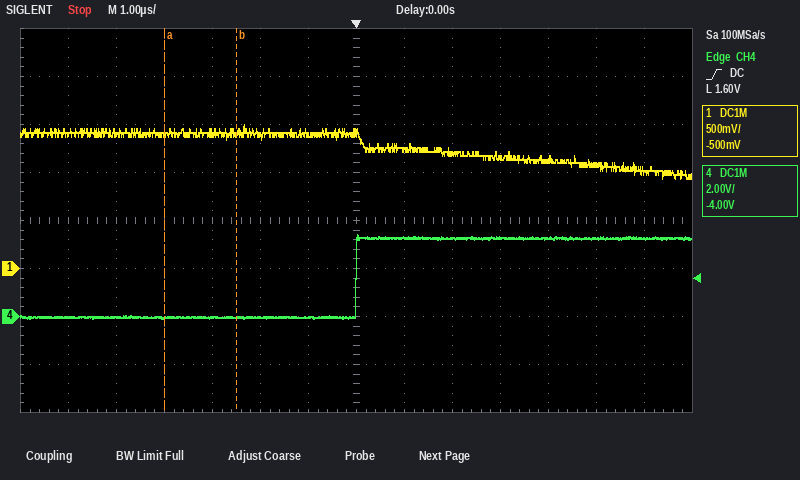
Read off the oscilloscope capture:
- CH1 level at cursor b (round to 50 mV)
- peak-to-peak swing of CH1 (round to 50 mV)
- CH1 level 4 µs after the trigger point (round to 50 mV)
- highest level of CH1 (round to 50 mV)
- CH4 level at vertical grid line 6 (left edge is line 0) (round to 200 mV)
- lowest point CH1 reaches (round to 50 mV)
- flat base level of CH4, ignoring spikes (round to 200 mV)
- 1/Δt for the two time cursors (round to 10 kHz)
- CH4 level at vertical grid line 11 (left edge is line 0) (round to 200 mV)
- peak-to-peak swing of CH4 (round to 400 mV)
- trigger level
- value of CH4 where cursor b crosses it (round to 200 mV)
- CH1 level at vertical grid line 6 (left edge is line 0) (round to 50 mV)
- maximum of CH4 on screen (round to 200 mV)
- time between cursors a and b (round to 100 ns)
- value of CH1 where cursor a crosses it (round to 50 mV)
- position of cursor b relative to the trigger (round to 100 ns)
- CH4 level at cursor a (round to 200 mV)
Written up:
1.40 V
550 mV
1.15 V
1.50 V
0.0 V
950 mV
0.0 V
670 kHz
3.2 V
3.6 V
1.60 V
0.0 V
1.40 V
3.4 V
1.5 µs
1.40 V
-2.5 µs
0.0 V
